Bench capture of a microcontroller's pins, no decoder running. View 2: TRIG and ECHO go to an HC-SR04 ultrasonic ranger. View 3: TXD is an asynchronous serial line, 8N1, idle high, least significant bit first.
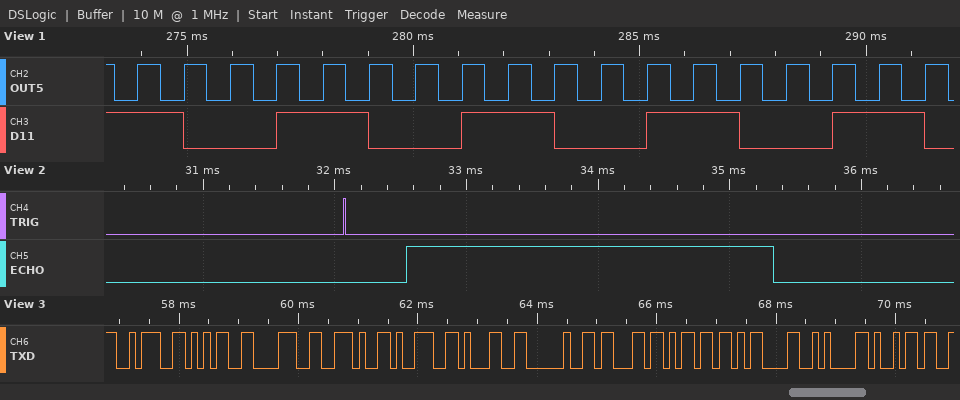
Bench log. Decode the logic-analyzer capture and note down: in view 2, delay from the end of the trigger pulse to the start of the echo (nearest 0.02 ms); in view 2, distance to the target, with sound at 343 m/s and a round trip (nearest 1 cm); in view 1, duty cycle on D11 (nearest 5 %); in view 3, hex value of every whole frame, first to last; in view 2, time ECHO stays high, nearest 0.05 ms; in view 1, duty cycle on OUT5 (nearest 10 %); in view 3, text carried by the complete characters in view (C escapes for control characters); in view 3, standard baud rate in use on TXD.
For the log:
0.46 ms
48 cm
50 %
0x3A 0x35 0x38 0x2E 0x39 0x31 0x20 0x63 0x6D 0x0D 0x0A 0x69
2.80 ms
50 %
":58.91 cm\r\ni"
9600 baud
